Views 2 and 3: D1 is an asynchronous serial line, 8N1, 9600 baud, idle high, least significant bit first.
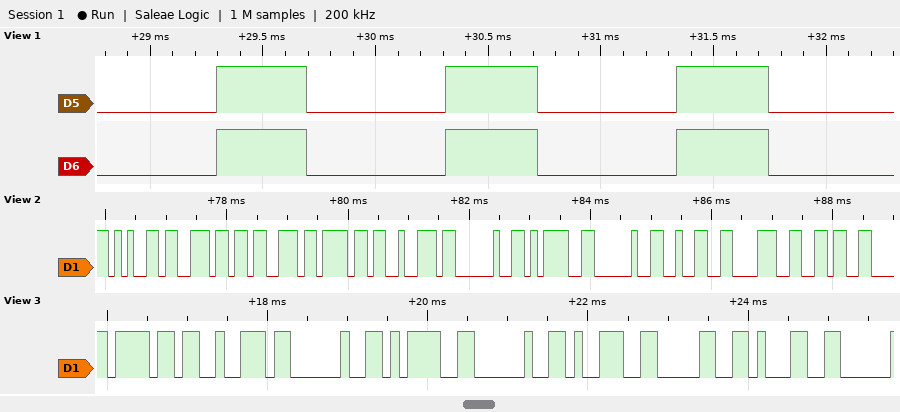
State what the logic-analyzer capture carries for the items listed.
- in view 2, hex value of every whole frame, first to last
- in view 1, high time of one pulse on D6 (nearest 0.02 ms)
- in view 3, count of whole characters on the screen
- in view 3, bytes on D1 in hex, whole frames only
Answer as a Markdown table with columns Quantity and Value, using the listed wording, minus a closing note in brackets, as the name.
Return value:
| Quantity | Value |
|---|---|
| in view 2, hex value of every whole frame, first to last | 0x65 0x6E 0x73 0x6F 0x72 0x20 0x3D 0x20 0x32 0x38 0x36 |
| in view 1, high time of one pulse on D6 | 0.40 ms |
| in view 3, count of whole characters on the screen | 8 |
| in view 3, bytes on D1 in hex, whole frames only | 6F 72 20 3D 20 39 30 31 |
